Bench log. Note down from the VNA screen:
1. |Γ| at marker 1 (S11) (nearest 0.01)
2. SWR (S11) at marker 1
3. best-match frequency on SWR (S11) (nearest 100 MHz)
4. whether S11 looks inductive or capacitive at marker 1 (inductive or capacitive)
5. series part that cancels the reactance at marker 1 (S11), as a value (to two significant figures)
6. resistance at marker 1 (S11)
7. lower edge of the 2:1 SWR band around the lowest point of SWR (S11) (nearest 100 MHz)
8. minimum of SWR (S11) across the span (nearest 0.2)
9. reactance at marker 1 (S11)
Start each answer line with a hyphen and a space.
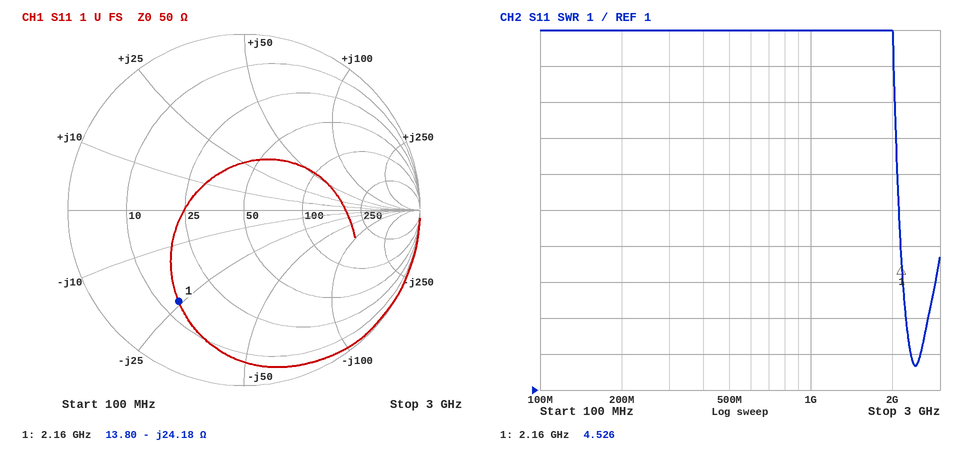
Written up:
- 0.64
- 4.526
- 2.4 GHz
- capacitive
- 1.8 nH
- 13.80 Ω
- 2.3 GHz
- 1.6
- -24.18 Ω
